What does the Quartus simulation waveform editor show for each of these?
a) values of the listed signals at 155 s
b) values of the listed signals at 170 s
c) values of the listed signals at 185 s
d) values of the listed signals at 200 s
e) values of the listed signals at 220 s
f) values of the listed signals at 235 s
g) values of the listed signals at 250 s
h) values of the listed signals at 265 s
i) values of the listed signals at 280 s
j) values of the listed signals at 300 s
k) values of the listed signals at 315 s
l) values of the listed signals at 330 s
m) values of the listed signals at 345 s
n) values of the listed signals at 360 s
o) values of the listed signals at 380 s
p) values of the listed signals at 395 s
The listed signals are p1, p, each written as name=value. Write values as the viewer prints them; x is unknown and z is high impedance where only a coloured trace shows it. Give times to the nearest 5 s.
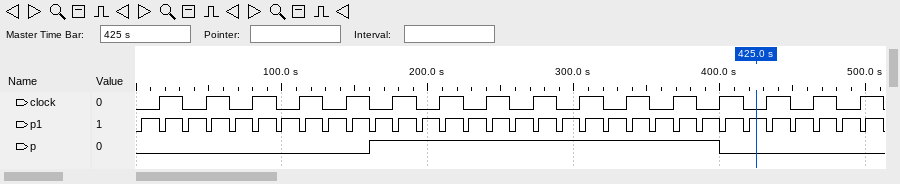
p1=1, p=0
p1=1, p=1
p1=1, p=1
p1=1, p=1
p1=1, p=1
p1=1, p=1
p1=1, p=1
p1=1, p=1
p1=1, p=1
p1=1, p=1
p1=1, p=1
p1=1, p=1
p1=1, p=1
p1=1, p=1
p1=1, p=1
p1=1, p=1
